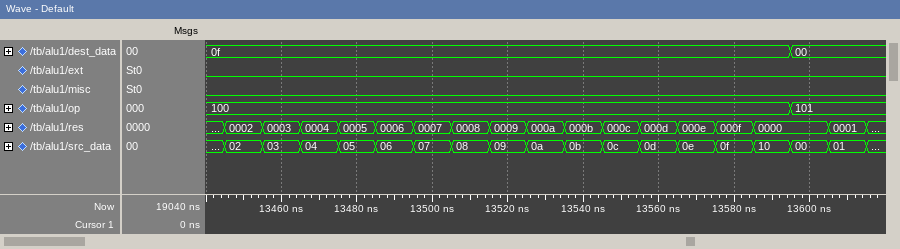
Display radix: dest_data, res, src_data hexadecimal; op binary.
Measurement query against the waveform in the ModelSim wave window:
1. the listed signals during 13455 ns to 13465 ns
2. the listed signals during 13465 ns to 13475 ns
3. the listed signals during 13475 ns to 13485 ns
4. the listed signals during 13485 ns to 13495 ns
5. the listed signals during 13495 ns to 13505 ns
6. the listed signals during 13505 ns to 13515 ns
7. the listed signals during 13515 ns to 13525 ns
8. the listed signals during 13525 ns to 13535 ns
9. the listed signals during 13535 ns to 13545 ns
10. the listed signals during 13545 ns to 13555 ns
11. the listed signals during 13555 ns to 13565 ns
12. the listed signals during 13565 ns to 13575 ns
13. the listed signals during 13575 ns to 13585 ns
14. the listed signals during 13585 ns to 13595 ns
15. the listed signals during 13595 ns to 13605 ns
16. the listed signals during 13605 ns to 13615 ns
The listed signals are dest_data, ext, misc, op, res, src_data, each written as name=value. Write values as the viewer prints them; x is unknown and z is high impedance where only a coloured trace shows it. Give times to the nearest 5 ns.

dest_data=0f, ext=0, misc=0, op=100, res=0003, src_data=03
dest_data=0f, ext=0, misc=0, op=100, res=0004, src_data=04
dest_data=0f, ext=0, misc=0, op=100, res=0005, src_data=05
dest_data=0f, ext=0, misc=0, op=100, res=0006, src_data=06
dest_data=0f, ext=0, misc=0, op=100, res=0007, src_data=07
dest_data=0f, ext=0, misc=0, op=100, res=0008, src_data=08
dest_data=0f, ext=0, misc=0, op=100, res=0009, src_data=09
dest_data=0f, ext=0, misc=0, op=100, res=000a, src_data=0a
dest_data=0f, ext=0, misc=0, op=100, res=000b, src_data=0b
dest_data=0f, ext=0, misc=0, op=100, res=000c, src_data=0c
dest_data=0f, ext=0, misc=0, op=100, res=000d, src_data=0d
dest_data=0f, ext=0, misc=0, op=100, res=000e, src_data=0e
dest_data=0f, ext=0, misc=0, op=100, res=000f, src_data=0f
dest_data=0f, ext=0, misc=0, op=100, res=0000, src_data=10
dest_data=00, ext=0, misc=0, op=101, res=0000, src_data=00
dest_data=00, ext=0, misc=0, op=101, res=0001, src_data=01
